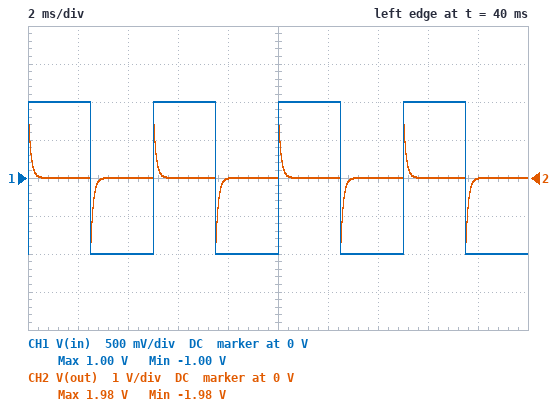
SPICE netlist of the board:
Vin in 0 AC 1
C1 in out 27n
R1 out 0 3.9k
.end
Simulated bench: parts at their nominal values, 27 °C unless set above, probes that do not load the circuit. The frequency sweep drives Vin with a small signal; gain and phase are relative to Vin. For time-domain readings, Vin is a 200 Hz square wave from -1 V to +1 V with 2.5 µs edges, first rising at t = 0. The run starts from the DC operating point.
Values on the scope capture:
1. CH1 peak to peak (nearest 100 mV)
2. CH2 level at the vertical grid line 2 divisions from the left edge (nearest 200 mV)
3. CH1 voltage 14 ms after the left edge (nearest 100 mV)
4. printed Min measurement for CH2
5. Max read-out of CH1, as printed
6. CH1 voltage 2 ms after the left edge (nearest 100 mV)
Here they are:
2.0 V
0 V
-1.0 V
-1.98 V
1.00 V
1.0 V
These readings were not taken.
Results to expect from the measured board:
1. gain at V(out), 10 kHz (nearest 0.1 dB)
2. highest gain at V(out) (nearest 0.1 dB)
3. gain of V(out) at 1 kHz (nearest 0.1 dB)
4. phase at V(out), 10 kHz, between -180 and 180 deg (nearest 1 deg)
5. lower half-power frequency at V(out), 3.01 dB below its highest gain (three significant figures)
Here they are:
-0.1 dB
0 dB
-5.2 dB
9 deg
1.51 kHz
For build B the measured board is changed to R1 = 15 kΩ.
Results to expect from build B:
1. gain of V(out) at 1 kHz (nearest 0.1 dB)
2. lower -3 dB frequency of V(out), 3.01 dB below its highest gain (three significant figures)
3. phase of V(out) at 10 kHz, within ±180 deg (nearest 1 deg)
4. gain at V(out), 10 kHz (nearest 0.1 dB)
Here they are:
-0.6 dB
393 Hz
2 deg
0 dB
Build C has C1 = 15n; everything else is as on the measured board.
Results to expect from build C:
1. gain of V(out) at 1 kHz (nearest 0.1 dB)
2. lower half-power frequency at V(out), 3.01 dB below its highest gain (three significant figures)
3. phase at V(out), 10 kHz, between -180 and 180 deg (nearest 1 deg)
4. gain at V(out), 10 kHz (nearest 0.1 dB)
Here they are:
-9.2 dB
2.72 kHz
15 deg
-0.3 dB
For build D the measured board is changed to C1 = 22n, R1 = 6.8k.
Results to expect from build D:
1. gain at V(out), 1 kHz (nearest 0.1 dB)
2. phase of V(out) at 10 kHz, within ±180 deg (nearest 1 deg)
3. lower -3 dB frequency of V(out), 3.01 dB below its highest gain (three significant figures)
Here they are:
-3.3 dB
6 deg
1.06 kHz
